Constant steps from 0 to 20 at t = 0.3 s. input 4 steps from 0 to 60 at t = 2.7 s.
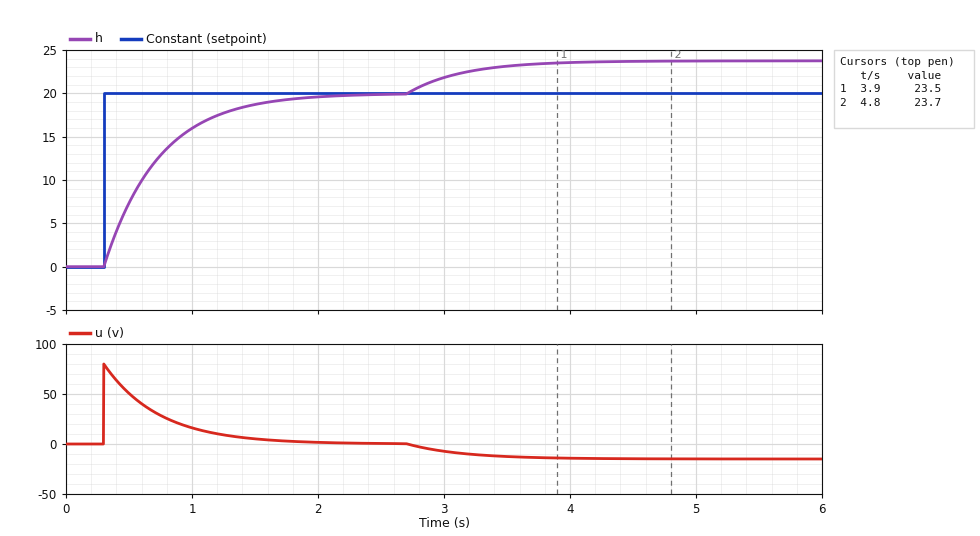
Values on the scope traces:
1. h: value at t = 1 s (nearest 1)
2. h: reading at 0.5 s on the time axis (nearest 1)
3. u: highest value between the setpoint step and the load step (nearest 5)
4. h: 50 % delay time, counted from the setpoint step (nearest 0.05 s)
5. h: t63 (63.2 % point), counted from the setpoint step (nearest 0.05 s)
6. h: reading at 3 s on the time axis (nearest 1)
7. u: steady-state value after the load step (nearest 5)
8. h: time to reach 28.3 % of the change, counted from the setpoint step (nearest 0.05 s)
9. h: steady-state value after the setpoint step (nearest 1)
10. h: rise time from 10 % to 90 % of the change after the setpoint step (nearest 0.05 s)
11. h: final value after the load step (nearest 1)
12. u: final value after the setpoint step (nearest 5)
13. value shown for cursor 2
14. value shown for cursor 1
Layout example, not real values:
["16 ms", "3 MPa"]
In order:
["16", "7", "80", "0.30 s", "0.45 s", "22", "-15", "0.15 s", "20", "0.95 s", "24", "0", "23.7", "23.5"]
